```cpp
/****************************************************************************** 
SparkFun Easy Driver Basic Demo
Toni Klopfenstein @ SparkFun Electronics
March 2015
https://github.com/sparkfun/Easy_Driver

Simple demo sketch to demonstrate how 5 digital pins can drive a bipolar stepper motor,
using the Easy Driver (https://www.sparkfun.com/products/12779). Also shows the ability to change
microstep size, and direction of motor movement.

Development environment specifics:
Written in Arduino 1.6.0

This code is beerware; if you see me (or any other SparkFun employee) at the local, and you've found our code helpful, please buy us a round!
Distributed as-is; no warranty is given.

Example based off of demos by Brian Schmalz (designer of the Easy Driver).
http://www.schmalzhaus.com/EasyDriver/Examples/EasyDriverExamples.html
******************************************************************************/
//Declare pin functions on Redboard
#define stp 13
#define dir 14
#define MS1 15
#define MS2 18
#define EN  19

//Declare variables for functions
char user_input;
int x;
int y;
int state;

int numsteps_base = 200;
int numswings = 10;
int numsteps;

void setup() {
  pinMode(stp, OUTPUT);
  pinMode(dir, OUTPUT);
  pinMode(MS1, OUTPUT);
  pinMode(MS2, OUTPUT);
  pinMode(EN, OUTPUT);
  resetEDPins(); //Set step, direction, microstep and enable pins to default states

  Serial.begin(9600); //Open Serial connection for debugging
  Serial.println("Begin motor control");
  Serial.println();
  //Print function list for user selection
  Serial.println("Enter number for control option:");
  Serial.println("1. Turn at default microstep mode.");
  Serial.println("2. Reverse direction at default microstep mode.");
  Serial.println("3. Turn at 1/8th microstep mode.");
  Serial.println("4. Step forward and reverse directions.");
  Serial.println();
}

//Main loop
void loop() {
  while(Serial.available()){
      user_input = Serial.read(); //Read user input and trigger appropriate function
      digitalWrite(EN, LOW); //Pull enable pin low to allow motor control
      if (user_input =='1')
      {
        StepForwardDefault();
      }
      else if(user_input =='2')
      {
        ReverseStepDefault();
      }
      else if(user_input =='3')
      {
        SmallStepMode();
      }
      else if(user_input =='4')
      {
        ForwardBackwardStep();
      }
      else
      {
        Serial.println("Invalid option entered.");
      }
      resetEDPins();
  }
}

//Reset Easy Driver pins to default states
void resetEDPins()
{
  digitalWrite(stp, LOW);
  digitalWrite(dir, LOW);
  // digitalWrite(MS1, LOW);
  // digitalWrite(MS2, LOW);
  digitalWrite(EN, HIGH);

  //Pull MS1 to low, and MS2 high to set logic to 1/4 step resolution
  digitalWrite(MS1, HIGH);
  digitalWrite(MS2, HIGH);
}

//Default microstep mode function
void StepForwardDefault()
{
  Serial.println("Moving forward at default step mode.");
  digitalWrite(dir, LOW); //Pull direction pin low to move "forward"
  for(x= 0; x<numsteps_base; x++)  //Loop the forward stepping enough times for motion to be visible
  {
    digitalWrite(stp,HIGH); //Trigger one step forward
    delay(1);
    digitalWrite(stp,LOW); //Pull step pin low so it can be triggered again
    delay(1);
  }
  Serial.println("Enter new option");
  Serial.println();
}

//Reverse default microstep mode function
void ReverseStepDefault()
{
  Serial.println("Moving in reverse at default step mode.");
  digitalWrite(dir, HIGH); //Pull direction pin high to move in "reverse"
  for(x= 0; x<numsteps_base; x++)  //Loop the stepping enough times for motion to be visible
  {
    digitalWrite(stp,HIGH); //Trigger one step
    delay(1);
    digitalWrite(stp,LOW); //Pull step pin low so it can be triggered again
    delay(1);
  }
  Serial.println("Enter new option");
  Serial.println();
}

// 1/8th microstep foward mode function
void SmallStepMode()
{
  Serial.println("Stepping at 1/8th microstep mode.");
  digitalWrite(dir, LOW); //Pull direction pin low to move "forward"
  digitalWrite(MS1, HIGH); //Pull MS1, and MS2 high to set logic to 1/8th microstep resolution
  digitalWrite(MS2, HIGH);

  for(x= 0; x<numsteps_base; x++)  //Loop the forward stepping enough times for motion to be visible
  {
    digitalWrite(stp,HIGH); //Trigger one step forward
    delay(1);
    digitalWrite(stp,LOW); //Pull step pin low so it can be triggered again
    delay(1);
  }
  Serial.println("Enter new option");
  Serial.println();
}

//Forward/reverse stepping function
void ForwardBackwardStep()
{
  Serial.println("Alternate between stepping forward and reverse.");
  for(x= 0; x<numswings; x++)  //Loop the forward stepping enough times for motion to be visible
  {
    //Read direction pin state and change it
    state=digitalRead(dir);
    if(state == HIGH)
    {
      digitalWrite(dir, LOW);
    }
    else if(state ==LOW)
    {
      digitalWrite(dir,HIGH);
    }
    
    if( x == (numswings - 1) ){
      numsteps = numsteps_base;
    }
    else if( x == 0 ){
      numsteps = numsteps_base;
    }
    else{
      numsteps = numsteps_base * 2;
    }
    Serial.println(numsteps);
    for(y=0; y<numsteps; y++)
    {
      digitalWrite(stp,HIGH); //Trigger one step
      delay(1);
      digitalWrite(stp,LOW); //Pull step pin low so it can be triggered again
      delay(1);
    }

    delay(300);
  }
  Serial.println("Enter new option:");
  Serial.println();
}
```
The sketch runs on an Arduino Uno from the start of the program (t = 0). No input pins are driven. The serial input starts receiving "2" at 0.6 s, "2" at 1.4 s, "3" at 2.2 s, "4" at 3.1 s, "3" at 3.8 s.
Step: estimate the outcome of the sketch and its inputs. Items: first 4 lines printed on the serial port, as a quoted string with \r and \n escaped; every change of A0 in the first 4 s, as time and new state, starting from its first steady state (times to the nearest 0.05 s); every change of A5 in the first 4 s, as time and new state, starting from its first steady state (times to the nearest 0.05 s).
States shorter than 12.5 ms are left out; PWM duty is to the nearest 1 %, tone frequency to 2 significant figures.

"Begin motor control\r\n\r\nEnter number for control option:\r\n1. Turn at default microstep mode.\r\n"
0 s low; 0.6 s high; 1 s low; 1.4 s high; 1.8 s low; 3.1 s high; 3.8 s low
0 s high; 0.6 s low; 1 s high; 1.4 s low; 1.8 s high; 2.2 s low; 2.6 s high; 3.1 s low
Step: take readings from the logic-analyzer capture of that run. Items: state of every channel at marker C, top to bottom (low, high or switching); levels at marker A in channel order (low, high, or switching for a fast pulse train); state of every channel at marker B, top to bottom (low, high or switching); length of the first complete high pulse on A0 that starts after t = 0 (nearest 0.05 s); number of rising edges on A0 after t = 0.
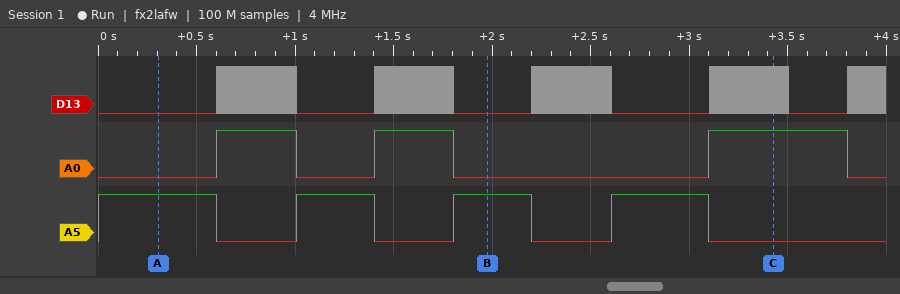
D13 switching, A0 high, A5 low
D13 low, A0 low, A5 high
D13 low, A0 low, A5 high
0.40 s
3
